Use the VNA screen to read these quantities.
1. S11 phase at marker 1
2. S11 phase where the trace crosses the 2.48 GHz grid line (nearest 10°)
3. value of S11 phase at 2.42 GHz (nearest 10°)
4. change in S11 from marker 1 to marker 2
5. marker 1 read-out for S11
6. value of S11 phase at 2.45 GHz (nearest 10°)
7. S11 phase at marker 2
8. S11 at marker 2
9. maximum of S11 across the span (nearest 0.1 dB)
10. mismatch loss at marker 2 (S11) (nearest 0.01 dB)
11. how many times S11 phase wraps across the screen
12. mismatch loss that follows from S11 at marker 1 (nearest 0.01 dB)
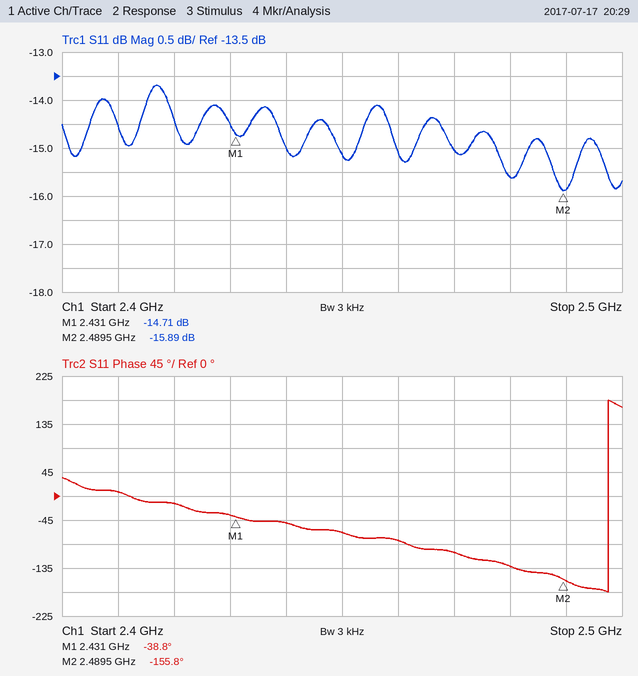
-38.8°
-130°
-10°
-1.18 dB
-14.71 dB
-70°
-155.8°
-15.89 dB
-13.7 dB
0.11 dB
1
0.15 dB
